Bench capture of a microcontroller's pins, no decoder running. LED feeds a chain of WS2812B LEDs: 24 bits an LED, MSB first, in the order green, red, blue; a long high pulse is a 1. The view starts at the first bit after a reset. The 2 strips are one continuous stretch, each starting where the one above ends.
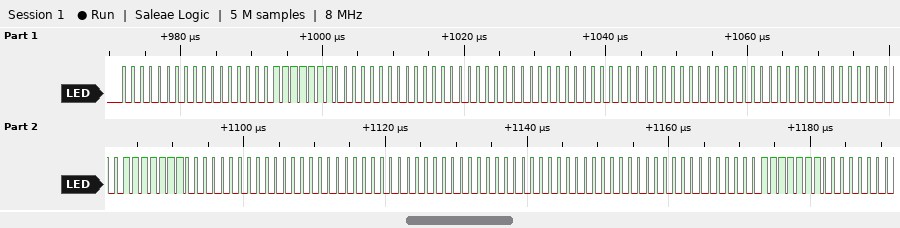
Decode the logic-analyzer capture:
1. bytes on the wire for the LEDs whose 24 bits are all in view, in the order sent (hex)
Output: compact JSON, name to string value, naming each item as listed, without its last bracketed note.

{"bytes on the wire for the LEDs whose 24 bits are all in view, in the order sent": "00 00 7F 00 00 00 00 00 00 00 00 7F 00 00 00 00 00 00 00 00 7F"}
